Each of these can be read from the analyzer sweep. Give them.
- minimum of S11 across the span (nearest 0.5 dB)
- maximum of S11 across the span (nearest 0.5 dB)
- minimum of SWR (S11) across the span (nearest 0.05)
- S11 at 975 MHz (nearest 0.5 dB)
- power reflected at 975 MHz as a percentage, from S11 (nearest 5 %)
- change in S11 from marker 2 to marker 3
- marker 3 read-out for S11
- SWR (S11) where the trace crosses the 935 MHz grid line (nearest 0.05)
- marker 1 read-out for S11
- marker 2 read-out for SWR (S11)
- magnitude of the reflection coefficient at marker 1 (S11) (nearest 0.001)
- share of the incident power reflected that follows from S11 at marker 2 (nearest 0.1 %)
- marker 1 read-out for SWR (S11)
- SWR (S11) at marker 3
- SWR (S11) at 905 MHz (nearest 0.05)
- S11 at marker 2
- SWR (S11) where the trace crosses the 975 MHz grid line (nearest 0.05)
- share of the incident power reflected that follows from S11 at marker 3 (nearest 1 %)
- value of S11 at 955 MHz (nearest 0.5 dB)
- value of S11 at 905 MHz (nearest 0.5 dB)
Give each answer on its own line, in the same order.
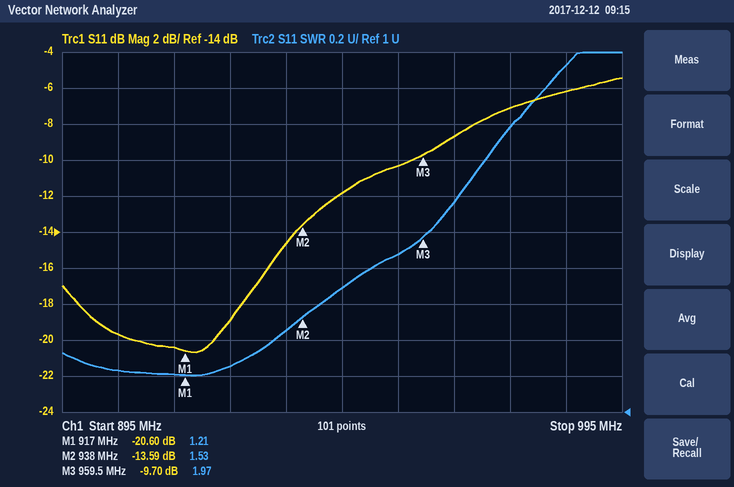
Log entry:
-20.5 dB
-5.5 dB
1.20
-7.0 dB
20 %
3.89 dB
-9.70 dB
1.45
-20.60 dB
1.53
0.093
4.4 %
1.21
1.97
1.25
-13.59 dB
2.60
11 %
-10.5 dB
-19.5 dB
